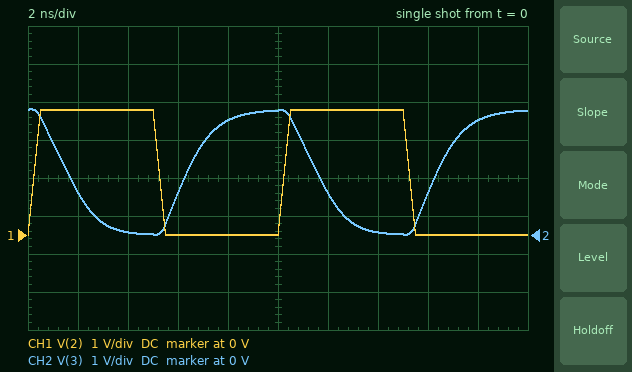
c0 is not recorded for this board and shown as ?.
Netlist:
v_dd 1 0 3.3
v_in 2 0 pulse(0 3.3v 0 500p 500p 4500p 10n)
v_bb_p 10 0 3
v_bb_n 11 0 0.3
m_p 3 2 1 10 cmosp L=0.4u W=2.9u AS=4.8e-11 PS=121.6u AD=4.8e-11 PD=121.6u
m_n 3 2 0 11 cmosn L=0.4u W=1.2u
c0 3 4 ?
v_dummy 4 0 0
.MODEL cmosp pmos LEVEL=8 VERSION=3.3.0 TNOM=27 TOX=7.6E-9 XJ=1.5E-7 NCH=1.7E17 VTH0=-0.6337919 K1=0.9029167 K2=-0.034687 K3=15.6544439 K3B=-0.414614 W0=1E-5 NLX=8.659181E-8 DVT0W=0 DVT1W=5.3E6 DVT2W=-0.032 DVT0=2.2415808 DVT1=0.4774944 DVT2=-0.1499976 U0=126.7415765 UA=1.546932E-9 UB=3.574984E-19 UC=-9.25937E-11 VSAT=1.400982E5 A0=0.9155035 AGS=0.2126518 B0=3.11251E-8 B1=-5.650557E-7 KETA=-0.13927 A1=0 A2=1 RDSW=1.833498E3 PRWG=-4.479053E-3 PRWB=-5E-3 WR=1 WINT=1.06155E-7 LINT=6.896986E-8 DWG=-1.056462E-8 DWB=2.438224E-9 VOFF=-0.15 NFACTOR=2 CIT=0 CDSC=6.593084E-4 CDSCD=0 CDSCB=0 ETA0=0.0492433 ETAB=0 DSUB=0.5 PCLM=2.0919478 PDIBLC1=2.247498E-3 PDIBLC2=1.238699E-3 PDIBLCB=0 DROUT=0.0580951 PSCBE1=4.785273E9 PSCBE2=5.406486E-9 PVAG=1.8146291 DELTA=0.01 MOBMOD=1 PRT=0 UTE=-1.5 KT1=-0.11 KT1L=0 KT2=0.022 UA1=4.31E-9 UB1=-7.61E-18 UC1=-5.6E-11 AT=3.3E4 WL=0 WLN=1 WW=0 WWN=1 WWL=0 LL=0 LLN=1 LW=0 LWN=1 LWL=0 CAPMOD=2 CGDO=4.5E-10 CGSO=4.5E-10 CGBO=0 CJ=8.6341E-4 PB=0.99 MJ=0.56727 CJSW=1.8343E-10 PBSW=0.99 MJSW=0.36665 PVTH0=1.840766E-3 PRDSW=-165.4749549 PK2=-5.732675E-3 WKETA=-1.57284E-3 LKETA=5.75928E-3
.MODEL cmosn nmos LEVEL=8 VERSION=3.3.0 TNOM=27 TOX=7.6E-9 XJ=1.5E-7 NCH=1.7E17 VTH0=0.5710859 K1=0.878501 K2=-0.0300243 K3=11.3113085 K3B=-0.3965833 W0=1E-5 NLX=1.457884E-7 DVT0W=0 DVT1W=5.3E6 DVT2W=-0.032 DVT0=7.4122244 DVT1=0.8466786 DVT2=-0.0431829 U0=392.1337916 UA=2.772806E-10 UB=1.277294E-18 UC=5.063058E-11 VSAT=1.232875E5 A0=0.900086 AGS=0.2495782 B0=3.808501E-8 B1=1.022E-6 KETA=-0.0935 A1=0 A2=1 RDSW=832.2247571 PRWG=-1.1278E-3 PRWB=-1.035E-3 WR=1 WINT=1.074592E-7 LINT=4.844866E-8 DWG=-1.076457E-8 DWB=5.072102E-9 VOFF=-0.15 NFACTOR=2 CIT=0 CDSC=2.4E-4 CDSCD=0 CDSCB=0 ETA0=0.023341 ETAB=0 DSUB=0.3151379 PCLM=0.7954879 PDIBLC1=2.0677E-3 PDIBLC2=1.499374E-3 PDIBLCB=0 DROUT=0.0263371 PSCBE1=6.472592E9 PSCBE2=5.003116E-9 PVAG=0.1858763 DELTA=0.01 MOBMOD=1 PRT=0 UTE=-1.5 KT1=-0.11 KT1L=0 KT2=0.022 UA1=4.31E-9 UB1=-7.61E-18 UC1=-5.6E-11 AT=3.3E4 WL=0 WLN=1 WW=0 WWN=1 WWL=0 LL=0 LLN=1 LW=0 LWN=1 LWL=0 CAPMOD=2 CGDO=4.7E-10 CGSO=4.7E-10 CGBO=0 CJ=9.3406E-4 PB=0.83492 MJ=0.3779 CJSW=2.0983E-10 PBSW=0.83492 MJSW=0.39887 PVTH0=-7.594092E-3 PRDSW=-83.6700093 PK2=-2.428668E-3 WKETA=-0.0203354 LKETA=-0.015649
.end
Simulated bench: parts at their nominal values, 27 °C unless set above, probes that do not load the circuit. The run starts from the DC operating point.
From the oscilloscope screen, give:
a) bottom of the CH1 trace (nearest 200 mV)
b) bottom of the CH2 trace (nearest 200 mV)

0 V
0 V
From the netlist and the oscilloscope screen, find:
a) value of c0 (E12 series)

390 fF
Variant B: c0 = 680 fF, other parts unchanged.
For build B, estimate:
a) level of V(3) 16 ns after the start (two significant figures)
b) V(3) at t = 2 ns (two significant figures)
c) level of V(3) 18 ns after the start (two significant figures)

830 mV
2.0 V
2.4 V
